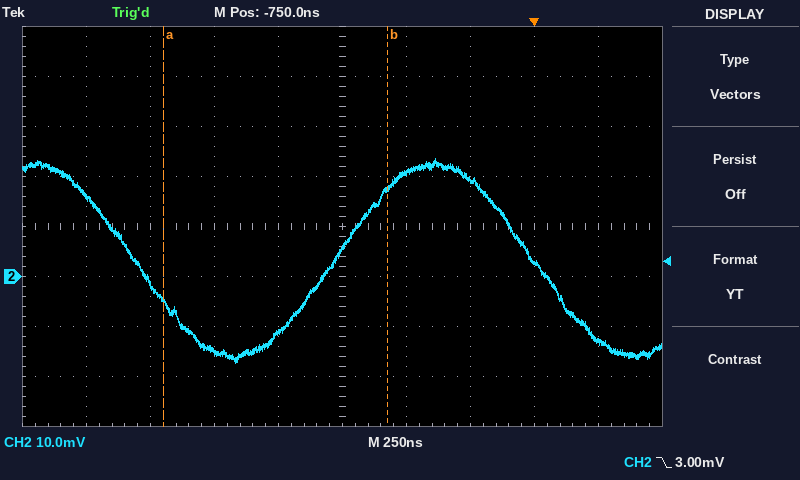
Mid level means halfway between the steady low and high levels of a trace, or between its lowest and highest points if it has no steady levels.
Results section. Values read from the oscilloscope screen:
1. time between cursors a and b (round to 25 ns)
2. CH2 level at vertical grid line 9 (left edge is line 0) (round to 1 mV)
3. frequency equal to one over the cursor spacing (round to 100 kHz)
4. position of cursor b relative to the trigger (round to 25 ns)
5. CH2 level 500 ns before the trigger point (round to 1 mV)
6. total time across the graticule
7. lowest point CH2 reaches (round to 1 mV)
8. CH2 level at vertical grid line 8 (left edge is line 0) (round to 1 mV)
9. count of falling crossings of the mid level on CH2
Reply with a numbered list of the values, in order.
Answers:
1. 875 ns
2. -13 mV
3. 1.1 MHz
4. -575 ns
5. 21 mV
6. 2.5 µs
7. -17 mV
8. 3 mV
9. 2
